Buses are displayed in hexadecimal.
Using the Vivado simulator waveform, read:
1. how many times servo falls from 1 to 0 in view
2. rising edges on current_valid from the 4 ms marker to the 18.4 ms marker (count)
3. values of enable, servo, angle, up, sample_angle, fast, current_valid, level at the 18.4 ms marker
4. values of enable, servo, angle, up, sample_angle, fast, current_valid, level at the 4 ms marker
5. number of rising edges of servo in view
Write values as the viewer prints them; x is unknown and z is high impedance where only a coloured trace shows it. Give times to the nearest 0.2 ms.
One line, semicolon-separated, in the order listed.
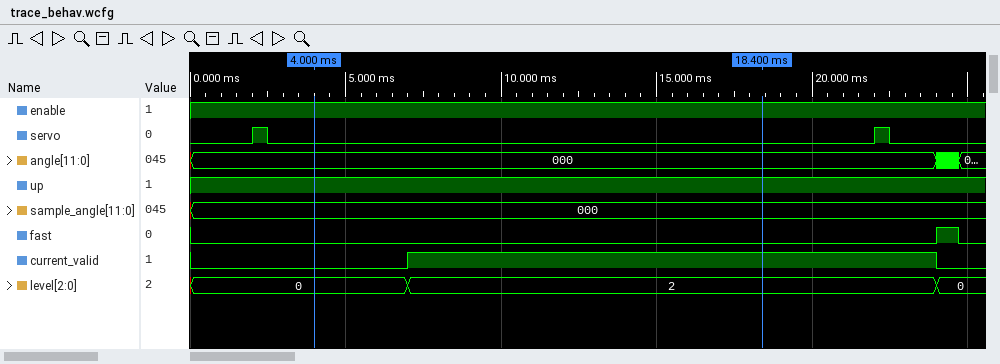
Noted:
2; 1; enable=1, servo=0, angle=000, up=1, sample_angle=000, fast=0, current_valid=1, level=2; enable=1, servo=0, angle=000, up=1, sample_angle=000, fast=0, current_valid=0, level=0; 2
